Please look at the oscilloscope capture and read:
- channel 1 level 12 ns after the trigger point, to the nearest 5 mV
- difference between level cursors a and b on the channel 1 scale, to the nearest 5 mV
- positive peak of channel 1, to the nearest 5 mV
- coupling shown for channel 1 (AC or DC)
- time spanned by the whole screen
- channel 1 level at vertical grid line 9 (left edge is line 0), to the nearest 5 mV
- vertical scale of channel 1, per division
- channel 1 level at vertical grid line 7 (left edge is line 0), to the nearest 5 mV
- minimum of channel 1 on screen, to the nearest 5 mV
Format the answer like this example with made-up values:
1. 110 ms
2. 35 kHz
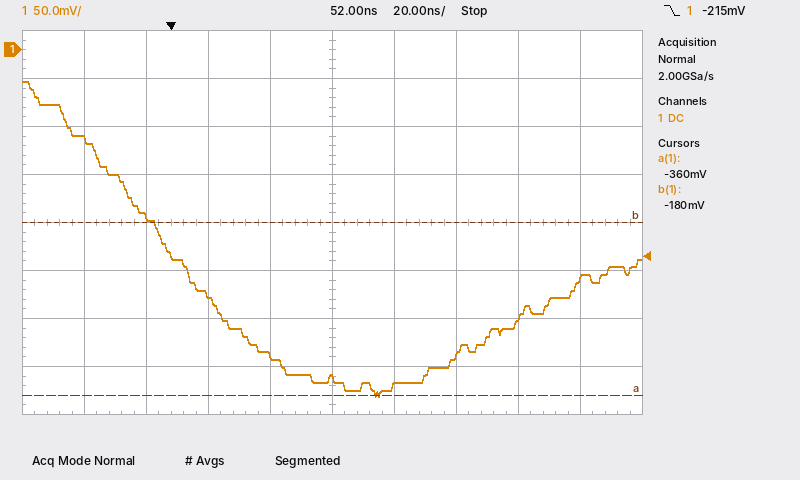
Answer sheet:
1. -255 mV
2. 180 mV
3. -35 mV
4. DC
5. 200 ns
6. -240 mV
7. 50 mV
8. -320 mV
9. -360 mV
